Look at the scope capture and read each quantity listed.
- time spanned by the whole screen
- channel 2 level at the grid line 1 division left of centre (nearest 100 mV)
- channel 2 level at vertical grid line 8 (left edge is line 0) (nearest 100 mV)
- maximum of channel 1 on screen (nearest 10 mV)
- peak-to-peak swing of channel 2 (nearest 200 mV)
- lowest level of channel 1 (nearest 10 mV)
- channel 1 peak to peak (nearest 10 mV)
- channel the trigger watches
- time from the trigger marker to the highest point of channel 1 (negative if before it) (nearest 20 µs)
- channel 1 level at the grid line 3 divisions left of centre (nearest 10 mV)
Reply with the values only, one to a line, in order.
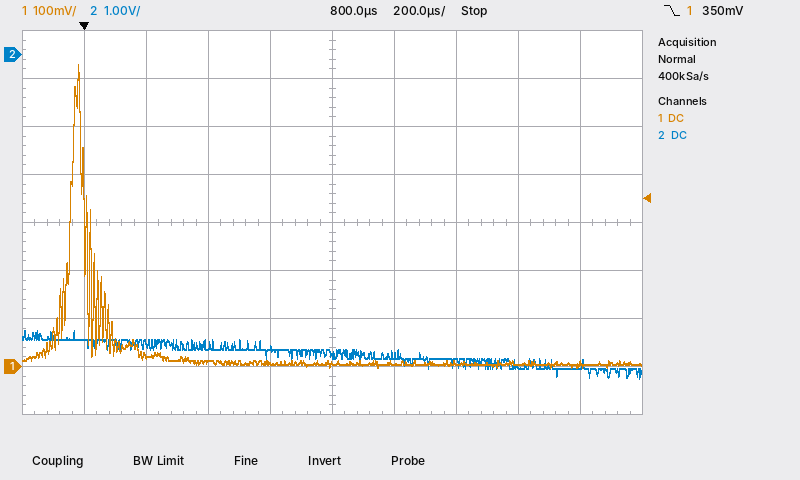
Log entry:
2 ms
-6.1 V
-6.5 V
630 mV
1.0 V
0 mV
630 mV
channel 1
-20 µs
20 mV
